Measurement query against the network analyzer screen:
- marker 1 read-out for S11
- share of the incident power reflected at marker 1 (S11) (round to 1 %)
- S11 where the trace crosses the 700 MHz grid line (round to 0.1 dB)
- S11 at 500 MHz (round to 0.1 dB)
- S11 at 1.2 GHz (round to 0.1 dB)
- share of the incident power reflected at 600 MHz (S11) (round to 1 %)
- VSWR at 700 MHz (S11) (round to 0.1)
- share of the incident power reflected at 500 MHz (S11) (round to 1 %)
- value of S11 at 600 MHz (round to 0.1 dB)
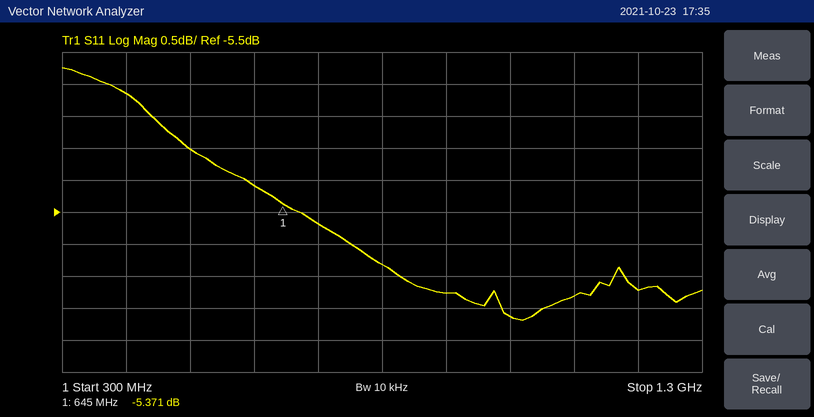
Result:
-5.371 dB
29 %
-5.7 dB
-4.5 dB
-6.7 dB
31 %
3.2
35 %
-5.1 dB
